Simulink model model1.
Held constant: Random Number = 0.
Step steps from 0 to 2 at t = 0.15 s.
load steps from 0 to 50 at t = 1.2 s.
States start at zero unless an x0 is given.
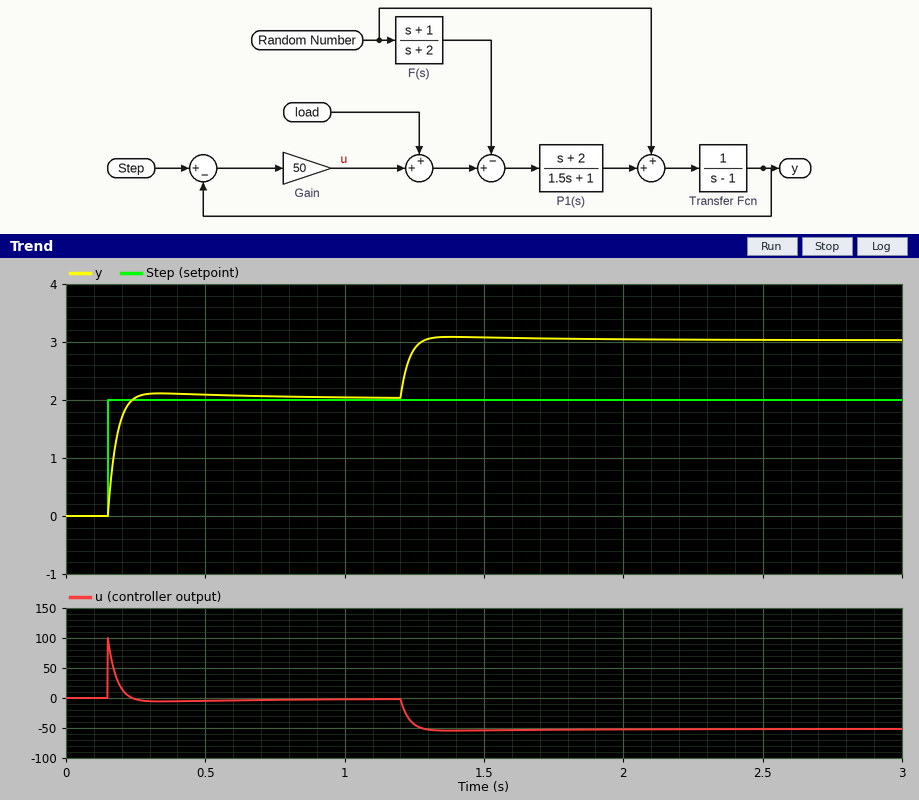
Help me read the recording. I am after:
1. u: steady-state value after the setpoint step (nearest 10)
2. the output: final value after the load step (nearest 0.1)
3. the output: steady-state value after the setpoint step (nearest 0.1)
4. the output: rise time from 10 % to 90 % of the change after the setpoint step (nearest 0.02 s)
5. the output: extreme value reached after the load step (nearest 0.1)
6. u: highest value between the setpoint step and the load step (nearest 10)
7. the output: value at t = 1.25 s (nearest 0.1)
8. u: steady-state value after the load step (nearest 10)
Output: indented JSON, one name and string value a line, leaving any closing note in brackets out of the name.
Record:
{
  "u: steady-state value after the setpoint step": "0",
  "the output: final value after the load step": "3.0",
  "the output: steady-state value after the setpoint step": "2.0",
  "the output: rise time from 10 % to 90 % of the change after the setpoint step": "0.06 s",
  "the output: extreme value reached after the load step": "3.1",
  "u: highest value between the setpoint step and the load step": "100",
  "the output: value at t = 1.25 s": "2.9",
  "u: steady-state value after the load step": "-50"
}
